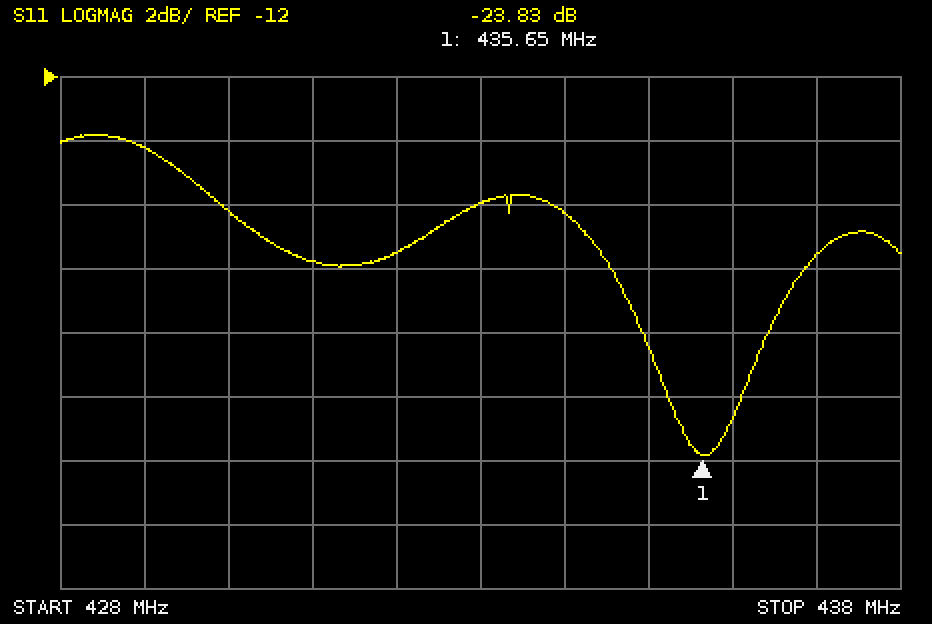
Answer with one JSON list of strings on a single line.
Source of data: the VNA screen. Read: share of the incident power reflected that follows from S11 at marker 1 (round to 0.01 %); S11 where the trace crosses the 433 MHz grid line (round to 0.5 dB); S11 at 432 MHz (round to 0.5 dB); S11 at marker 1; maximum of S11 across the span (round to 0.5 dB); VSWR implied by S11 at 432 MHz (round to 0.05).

["0.41 %", "-16.0 dB", "-17.5 dB", "-23.83 dB", "-14.0 dB", "1.30"]
